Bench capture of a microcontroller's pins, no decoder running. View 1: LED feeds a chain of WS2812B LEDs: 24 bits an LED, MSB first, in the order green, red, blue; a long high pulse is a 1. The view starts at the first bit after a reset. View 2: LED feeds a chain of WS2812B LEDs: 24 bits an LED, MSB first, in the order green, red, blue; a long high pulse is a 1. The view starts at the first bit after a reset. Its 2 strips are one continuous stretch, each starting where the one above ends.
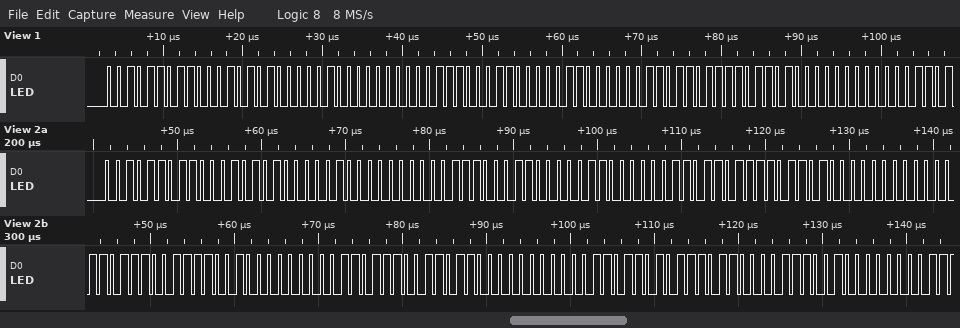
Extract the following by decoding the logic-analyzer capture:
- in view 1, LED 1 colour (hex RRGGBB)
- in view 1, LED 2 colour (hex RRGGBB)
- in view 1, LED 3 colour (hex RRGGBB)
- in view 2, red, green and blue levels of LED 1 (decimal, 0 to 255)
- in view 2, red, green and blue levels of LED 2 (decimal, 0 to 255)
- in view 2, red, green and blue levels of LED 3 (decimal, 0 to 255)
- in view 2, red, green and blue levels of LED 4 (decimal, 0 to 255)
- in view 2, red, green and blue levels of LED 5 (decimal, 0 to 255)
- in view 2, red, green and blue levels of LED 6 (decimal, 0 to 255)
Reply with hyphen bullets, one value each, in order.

- #8A2D82
- #710083
- #6F0368
- 138, 45, 130
- 113, 0, 131
- 111, 3, 104
- 110, 0, 121
- 110, 0, 108
- 109, 0, 118
